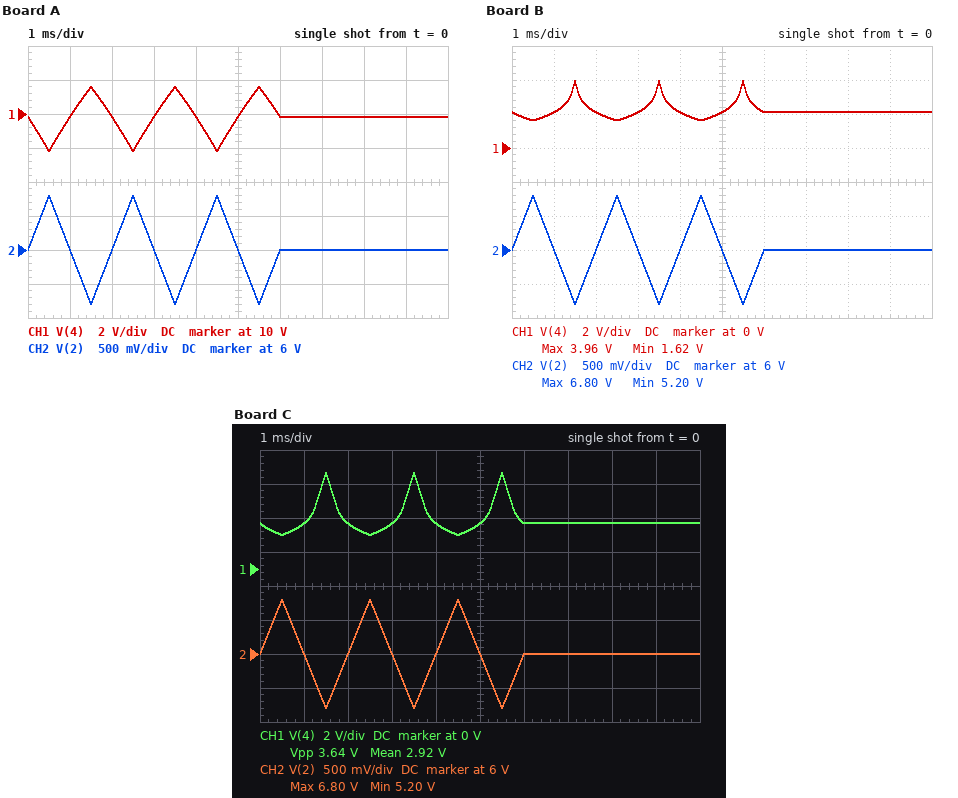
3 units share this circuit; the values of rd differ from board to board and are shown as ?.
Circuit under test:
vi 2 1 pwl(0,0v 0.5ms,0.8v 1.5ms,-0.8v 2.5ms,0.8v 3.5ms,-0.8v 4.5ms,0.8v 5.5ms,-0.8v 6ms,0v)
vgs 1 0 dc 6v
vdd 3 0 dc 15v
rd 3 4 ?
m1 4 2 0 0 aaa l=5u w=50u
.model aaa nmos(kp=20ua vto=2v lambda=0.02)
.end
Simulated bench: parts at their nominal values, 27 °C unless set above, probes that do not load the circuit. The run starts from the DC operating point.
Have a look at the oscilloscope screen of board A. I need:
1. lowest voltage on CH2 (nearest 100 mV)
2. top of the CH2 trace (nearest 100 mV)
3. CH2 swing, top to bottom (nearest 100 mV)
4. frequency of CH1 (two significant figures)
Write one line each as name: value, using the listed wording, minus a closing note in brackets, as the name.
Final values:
lowest voltage on CH2: 5.2 V
top of the CH2 trace: 6.8 V
CH2 swing, top to bottom: 1.6 V
frequency of CH1: 500 Hz
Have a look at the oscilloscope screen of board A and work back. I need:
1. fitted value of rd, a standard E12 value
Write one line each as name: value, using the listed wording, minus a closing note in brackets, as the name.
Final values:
fitted value of rd, a standard E12 value: 2.7 kΩ
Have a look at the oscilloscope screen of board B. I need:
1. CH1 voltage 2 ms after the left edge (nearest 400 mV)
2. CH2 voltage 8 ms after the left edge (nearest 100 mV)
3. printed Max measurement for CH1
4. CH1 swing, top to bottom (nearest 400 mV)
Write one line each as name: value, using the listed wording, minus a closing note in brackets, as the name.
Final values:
CH1 voltage 2 ms after the left edge: 2.0 V
CH2 voltage 8 ms after the left edge: 6.0 V
printed Max measurement for CH1: 3.96 V
CH1 swing, top to bottom: 2.4 V
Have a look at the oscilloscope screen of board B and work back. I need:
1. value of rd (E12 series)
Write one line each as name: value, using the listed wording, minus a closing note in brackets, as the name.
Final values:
value of rd: 10 kΩ
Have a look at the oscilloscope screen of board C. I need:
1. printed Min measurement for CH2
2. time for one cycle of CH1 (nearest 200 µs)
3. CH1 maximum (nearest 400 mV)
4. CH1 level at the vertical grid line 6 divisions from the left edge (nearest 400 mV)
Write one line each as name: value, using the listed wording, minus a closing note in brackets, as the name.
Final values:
printed Min measurement for CH2: 5.20 V
time for one cycle of CH1: 2.0 ms
CH1 maximum: 5.6 V
CH1 level at the vertical grid line 6 divisions from the left edge: 2.8 V
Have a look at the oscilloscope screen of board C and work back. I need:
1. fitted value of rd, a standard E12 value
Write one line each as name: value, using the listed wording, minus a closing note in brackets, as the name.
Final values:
fitted value of rd, a standard E12 value: 8.2 kΩ
